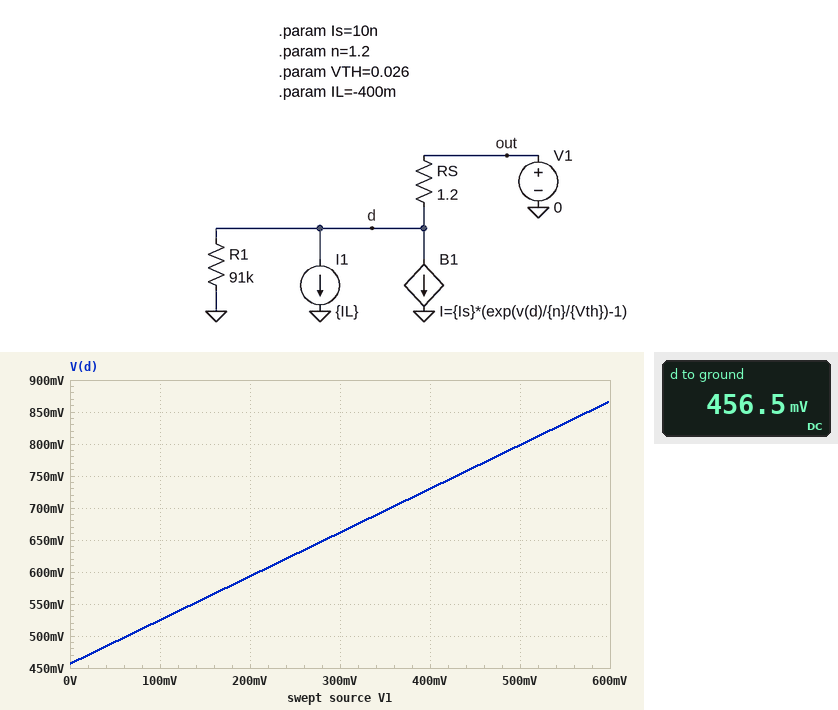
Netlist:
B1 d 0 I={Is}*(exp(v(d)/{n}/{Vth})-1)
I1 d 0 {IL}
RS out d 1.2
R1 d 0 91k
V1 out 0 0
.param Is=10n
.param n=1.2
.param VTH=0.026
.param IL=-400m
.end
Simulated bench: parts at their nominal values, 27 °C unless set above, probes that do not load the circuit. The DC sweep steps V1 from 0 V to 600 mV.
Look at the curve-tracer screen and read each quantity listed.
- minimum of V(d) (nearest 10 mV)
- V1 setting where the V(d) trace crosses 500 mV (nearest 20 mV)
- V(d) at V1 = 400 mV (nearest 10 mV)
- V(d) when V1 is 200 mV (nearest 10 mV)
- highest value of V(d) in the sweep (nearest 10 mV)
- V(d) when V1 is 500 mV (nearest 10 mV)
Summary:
460 mV
60 mV
730 mV
590 mV
870 mV
800 mV
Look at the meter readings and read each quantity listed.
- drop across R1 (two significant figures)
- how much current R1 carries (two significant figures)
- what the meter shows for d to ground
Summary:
460 mV
5.0 µA
456.5 mV
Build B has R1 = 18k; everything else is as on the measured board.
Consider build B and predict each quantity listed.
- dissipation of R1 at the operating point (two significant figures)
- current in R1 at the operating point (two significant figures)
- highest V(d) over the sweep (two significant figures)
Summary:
12 µW
25 µA
870 mV
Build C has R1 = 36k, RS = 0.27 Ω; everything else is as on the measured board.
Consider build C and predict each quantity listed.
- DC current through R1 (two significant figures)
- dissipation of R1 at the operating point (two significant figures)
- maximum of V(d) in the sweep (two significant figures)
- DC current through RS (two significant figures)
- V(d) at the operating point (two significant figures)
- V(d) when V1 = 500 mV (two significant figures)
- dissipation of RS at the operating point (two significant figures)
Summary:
3.0 µA
320 nW
680 mV
400 mA
110 mV
590 mV
43 mW
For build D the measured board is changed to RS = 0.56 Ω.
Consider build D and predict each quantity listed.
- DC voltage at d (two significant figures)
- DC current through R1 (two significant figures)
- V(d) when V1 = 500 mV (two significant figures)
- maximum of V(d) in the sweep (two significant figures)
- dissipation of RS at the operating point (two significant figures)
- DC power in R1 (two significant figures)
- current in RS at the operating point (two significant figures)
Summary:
220 mV
2.5 µA
670 mV
750 mV
90 mW
550 nW
400 mA
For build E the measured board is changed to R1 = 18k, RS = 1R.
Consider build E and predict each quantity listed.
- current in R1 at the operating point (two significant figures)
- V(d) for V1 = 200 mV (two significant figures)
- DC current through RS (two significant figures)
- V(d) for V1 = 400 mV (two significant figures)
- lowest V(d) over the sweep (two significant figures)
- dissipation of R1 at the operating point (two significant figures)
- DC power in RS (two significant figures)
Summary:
22 µA
550 mV
400 mA
690 mV
400 mV
8.7 µW
160 mW
